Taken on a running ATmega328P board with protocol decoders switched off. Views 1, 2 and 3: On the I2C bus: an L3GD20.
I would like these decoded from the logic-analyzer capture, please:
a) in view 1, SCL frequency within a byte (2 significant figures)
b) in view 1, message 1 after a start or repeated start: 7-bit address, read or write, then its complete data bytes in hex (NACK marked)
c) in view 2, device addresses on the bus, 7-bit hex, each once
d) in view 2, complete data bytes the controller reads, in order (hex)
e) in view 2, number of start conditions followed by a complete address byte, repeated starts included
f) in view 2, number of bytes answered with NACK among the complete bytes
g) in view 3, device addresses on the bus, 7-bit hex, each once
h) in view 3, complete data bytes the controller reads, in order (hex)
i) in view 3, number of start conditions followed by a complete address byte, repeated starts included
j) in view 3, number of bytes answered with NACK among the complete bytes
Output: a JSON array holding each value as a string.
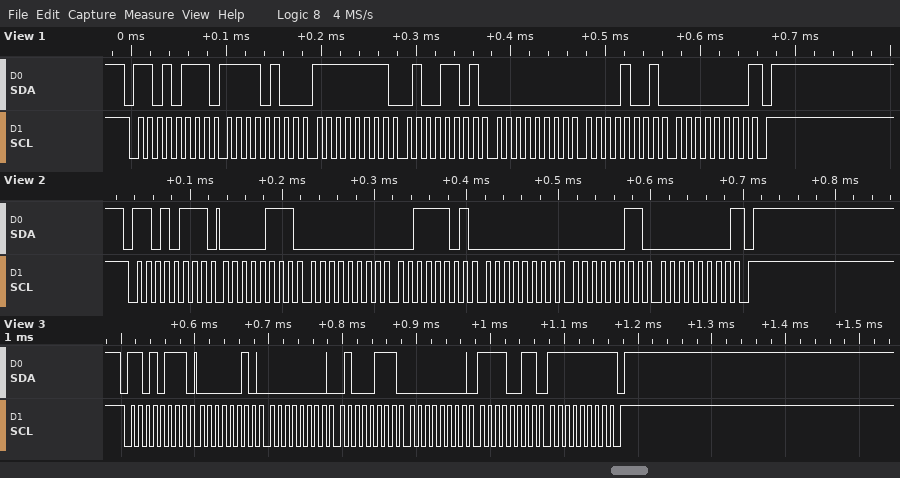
["100 kHz", "0x6B read: F4 FF 4D 00 09 00 NACK", "0x6B", "07 00 3D 00 03 00", "1", "1", "0x6B", "02 00 47 00 F3 FF", "1", "1"]
